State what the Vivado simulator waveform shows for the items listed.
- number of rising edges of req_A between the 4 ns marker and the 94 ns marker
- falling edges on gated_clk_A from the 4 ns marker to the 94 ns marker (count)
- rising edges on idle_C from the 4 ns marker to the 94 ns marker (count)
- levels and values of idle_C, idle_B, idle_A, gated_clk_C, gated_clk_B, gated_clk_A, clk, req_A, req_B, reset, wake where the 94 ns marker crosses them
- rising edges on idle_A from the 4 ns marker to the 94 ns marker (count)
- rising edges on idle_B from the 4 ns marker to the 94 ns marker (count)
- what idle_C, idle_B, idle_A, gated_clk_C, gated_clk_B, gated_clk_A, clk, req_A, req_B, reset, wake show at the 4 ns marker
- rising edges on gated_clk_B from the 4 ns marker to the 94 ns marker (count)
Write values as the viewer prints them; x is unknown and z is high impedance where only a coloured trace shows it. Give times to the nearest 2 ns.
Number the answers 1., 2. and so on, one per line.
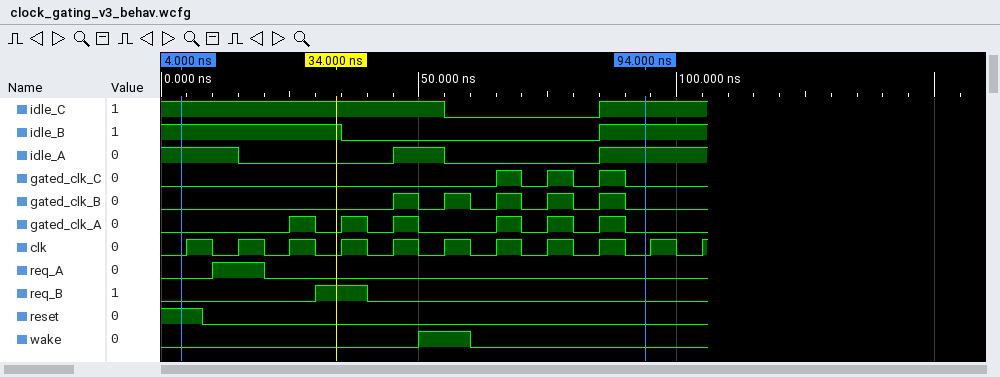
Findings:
1. 1
2. 6
3. 1
4. idle_C=1, idle_B=1, idle_A=1, gated_clk_C=0, gated_clk_B=0, gated_clk_A=0, clk=0, req_A=0, req_B=0, reset=0, wake=0
5. 2
6. 1
7. idle_C=1, idle_B=1, idle_A=1, gated_clk_C=0, gated_clk_B=0, gated_clk_A=0, clk=0, req_A=0, req_B=0, reset=1, wake=0
8. 5
